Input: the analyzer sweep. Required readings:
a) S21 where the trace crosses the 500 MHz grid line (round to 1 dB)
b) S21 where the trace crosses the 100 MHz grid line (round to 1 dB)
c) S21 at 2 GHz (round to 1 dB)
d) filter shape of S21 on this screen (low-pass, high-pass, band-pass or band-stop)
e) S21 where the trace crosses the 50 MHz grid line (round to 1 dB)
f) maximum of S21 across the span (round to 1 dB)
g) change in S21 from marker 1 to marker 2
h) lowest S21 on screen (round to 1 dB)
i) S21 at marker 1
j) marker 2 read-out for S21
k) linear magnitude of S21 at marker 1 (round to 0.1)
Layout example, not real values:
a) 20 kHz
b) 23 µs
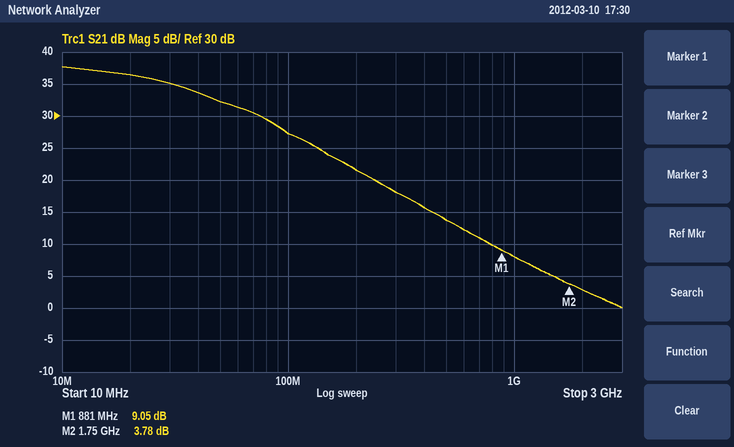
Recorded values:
a) 14 dB
b) 27 dB
c) 3 dB
d) low-pass
e) 32 dB
f) 38 dB
g) -5.27 dB
h) 0 dB
i) 9.05 dB
j) 3.78 dB
k) 2.8
